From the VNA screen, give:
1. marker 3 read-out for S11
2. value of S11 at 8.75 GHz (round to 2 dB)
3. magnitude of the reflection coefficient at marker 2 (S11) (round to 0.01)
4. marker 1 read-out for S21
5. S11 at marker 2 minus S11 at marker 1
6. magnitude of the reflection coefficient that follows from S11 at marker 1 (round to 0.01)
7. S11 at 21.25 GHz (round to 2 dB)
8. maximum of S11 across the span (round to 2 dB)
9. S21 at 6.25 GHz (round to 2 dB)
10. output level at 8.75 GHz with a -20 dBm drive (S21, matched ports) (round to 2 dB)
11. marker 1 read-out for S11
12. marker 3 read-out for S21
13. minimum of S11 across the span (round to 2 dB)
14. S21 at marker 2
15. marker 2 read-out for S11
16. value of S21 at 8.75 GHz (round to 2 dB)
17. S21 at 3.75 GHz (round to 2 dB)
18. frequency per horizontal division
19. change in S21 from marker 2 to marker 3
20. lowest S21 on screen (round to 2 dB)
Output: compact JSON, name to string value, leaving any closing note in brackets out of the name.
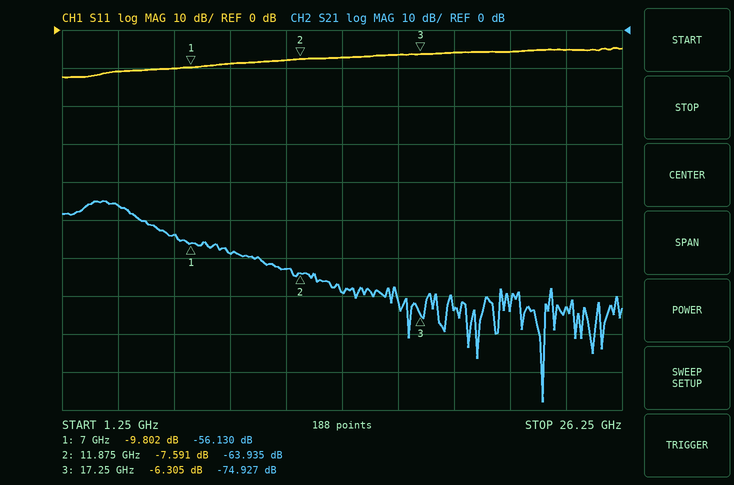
{"marker 3 read-out for S11": "-6.305 dB", "value of S11 at 8.75 GHz": "-8 dB", "magnitude of the reflection coefficient at marker 2 (S11)": "0.42", "marker 1 read-out for S21": "-56.130 dB", "S11 at marker 2 minus S11 at marker 1": "2.211 dB", "magnitude of the reflection coefficient that follows from S11 at marker 1": "0.32", "S11 at 21.25 GHz": "-6 dB", "maximum of S11 across the span": "-4 dB", "S21 at 6.25 GHz": "-54 dB", "output level at 8.75 GHz with a -20 dBm drive (S21, matched ports)": "-78 dBm", "marker 1 read-out for S11": "-9.802 dB", "marker 3 read-out for S21": "-74.927 dB", "minimum of S11 across the span": "-12 dB", "S21 at marker 2": "-63.935 dB", "marker 2 read-out for S11": "-7.591 dB", "value of S21 at 8.75 GHz": "-58 dB", "S21 at 3.75 GHz": "-46 dB", "frequency per horizontal division": "2.5 GHz", "change in S21 from marker 2 to marker 3": "-10.992 dB", "lowest S21 on screen": "-98 dB"}
